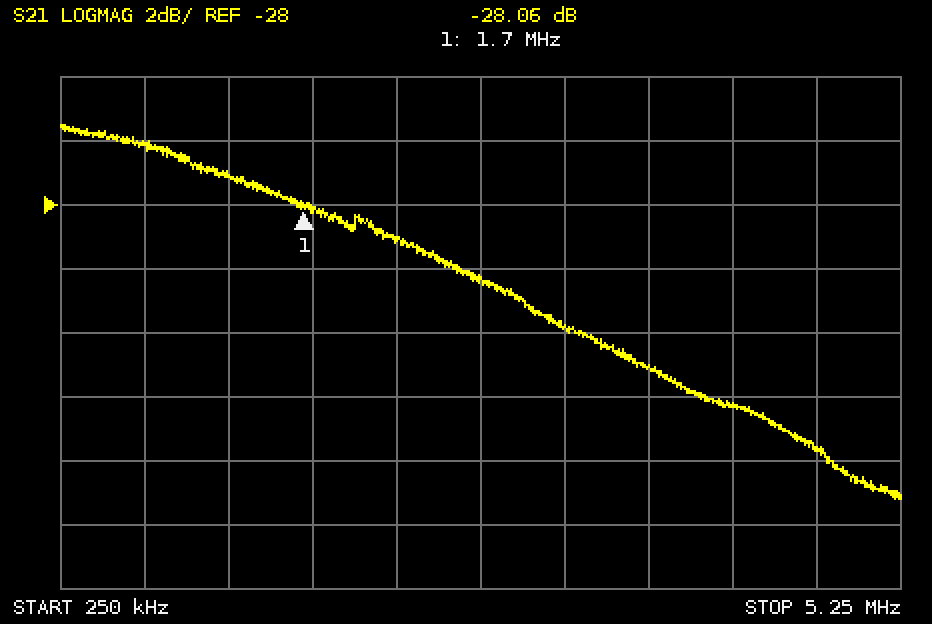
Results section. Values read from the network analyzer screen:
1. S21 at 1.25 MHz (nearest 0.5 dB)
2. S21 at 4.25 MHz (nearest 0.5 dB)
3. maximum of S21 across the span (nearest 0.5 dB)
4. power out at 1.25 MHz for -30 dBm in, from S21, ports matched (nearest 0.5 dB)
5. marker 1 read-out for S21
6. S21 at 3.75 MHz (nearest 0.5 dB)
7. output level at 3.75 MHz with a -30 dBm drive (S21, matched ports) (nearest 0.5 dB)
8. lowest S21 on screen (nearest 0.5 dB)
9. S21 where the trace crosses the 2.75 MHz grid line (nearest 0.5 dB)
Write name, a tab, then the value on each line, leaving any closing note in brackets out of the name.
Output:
S21 at 1.25 MHz	-27.0 dB
S21 at 4.25 MHz	-34.5 dB
maximum of S21 across the span	-25.5 dB
power out at 1.25 MHz for -30 dBm in, from S21, ports matched	-57.0 dBm
marker 1 read-out for S21	-28.06 dB
S21 at 3.75 MHz	-33.0 dB
output level at 3.75 MHz with a -30 dBm drive (S21, matched ports)	-63.0 dBm
lowest S21 on screen	-37.0 dB
S21 where the trace crosses the 2.75 MHz grid line	-30.5 dB
